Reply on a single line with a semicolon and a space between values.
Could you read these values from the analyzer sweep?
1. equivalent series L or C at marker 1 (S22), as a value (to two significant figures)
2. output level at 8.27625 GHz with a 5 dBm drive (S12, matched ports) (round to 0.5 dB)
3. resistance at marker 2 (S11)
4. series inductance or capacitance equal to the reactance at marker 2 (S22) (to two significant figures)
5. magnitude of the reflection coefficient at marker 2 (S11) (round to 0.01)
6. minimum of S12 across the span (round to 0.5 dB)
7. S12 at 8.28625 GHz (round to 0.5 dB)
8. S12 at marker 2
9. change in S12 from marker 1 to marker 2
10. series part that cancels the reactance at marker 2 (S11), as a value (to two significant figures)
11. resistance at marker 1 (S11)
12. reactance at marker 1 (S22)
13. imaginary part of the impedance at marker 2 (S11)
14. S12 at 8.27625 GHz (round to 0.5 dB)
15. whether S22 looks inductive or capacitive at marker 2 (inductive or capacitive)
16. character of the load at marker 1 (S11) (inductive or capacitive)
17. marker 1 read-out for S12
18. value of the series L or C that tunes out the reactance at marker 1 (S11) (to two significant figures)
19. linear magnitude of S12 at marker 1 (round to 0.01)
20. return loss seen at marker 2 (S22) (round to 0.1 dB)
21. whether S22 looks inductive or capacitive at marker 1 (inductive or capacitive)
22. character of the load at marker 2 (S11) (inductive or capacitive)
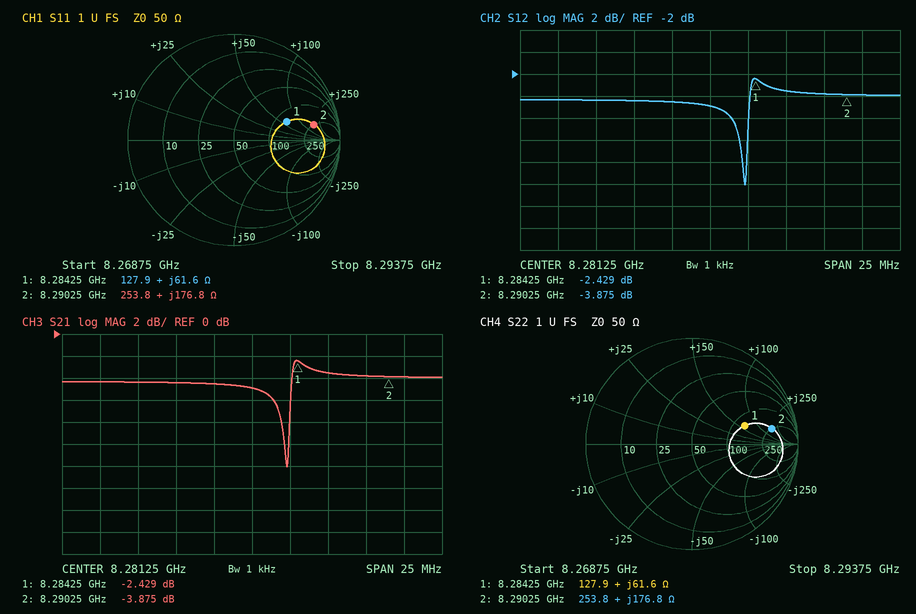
1.2 nH; 0.5 dBm; 253.8 Ω; 3.4 nH; 0.77; -12.0 dB; -3.5 dB; -3.875 dB; -1.446 dB; 110 fF; 127.9 Ω; +61.6 Ω; +176.8 Ω; -4.5 dB; inductive; inductive; -2.429 dB; 310 fF; 0.76; 2.3 dB; inductive; inductive
